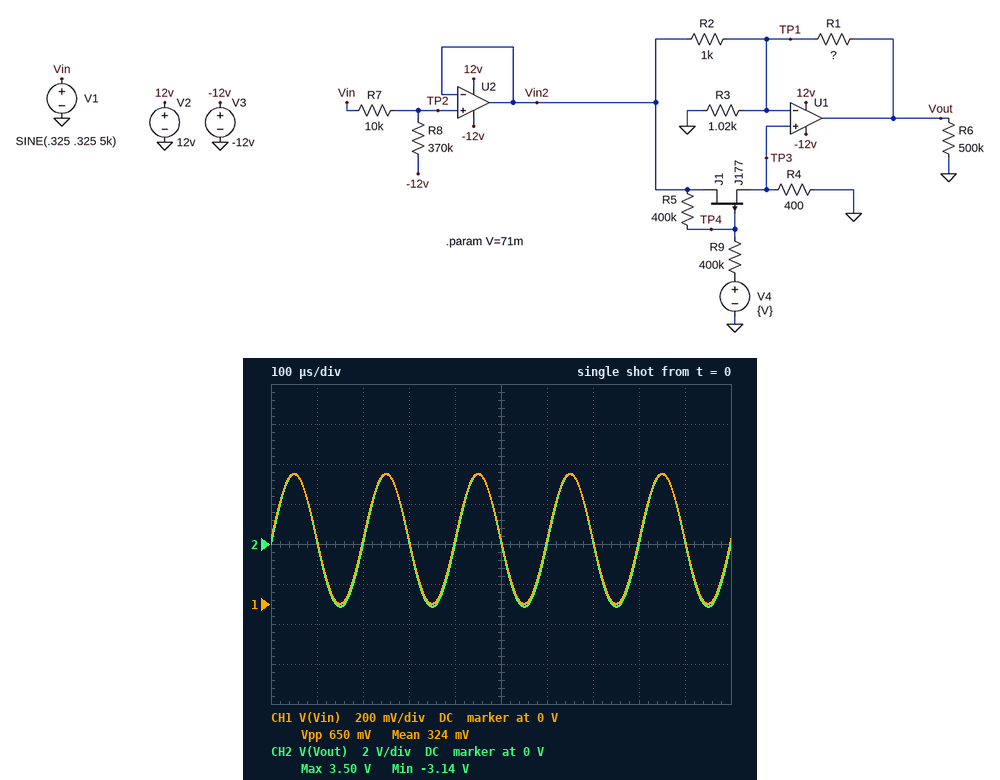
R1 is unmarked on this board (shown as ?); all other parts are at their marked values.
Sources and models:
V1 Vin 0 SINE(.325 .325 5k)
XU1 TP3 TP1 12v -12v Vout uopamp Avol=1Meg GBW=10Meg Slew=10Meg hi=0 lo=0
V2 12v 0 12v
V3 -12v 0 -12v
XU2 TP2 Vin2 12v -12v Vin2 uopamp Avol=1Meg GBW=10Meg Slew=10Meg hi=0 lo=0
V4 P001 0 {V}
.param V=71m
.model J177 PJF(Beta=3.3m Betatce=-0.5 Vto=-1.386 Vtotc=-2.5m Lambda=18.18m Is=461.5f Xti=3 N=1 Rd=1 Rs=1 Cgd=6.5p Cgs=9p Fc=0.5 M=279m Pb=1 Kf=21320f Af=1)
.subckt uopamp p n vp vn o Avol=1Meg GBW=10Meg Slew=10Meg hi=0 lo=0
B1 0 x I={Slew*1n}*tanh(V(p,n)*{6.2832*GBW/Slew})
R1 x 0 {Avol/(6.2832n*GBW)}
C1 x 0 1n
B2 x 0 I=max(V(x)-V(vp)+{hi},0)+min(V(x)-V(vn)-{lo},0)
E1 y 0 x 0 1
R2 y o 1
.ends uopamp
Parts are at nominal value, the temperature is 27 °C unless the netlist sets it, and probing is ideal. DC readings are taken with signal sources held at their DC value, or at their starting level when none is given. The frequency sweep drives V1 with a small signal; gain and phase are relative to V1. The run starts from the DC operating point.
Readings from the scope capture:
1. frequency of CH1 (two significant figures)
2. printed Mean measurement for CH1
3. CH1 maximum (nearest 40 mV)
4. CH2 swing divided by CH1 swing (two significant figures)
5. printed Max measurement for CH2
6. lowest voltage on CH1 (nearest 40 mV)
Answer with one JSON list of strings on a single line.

["5.0 kHz", "324 mV", "640 mV", "10", "3.50 V", "0 V"]
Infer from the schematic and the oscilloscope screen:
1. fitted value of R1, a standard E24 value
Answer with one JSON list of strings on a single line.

["18 kΩ"]
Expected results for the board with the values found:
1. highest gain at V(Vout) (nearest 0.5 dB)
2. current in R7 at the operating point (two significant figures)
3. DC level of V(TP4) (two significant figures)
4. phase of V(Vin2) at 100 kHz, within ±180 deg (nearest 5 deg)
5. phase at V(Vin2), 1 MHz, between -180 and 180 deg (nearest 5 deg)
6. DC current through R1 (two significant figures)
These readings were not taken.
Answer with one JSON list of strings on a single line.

["20.0 dB", "32 µA", "36 mV", "0 deg", "-5 deg", "360 nA"]
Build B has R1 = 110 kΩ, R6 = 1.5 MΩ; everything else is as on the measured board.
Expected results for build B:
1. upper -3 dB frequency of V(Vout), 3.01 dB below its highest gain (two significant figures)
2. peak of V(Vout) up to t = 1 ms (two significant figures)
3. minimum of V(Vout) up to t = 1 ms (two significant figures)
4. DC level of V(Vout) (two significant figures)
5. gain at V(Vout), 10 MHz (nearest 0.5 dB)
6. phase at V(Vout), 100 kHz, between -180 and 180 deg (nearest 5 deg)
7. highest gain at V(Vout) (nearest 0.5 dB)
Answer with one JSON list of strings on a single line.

["46 kHz", "12 V", "-12 V", "40 mV", "-14.5 dB", "-65 deg", "35.5 dB"]
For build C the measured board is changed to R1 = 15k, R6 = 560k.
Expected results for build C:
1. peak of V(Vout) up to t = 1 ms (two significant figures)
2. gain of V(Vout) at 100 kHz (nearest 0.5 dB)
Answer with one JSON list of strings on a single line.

["3.0 V", "18.5 dB"]
